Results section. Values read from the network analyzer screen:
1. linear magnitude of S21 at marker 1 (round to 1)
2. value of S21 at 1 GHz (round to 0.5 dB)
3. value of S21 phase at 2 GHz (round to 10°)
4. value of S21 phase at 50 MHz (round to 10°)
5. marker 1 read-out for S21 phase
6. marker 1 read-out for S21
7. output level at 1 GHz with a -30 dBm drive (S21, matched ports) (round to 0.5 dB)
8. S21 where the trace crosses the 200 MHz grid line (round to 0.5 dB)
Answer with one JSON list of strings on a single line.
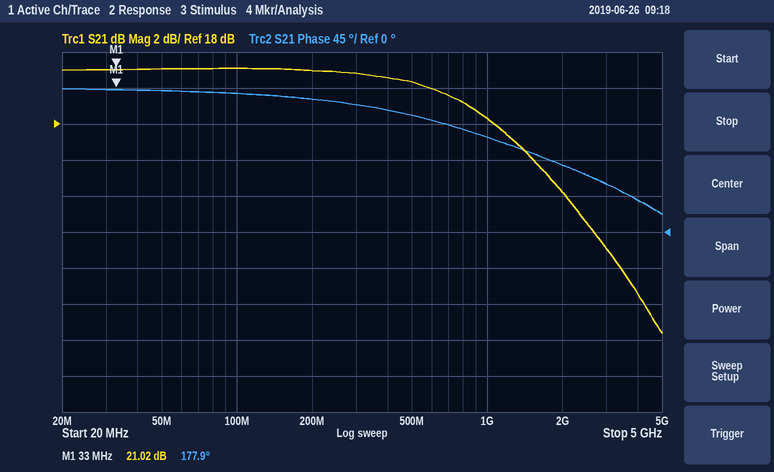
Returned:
["11", "18.5 dB", "80°", "180°", "177.9°", "21.02 dB", "-11.5 dBm", "21.0 dB"]
